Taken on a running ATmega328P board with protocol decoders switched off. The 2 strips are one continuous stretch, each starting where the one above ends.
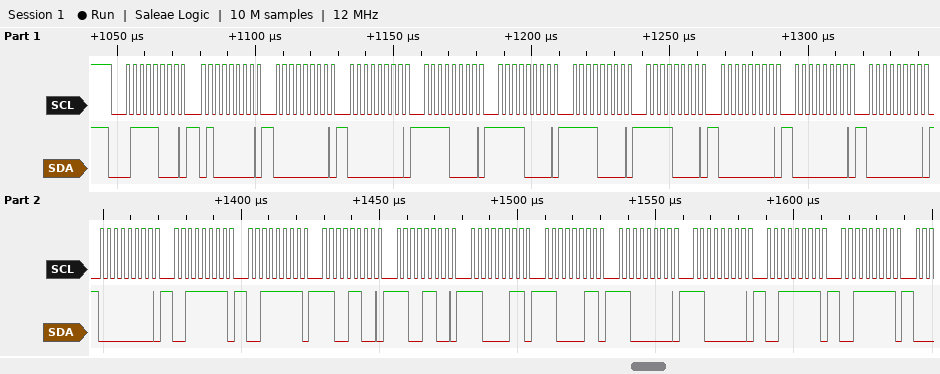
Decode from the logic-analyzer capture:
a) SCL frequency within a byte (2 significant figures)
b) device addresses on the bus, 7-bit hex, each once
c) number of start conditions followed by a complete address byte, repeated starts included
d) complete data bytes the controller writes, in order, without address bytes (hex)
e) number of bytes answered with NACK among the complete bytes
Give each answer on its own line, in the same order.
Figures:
400 kHz
0x3C
1
40 00 00 F0 F0 F0 F0 00 00 00 00 3F 3F CC CC C3 C3 C0 C0 3F 3F
0
